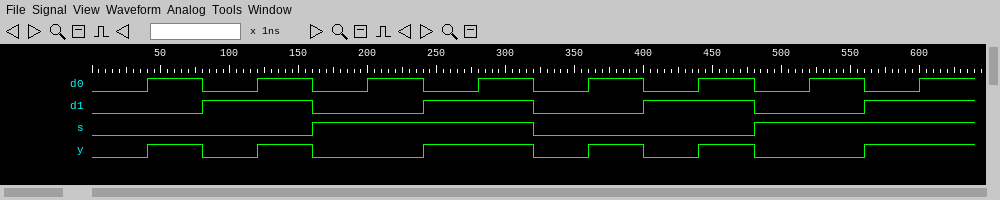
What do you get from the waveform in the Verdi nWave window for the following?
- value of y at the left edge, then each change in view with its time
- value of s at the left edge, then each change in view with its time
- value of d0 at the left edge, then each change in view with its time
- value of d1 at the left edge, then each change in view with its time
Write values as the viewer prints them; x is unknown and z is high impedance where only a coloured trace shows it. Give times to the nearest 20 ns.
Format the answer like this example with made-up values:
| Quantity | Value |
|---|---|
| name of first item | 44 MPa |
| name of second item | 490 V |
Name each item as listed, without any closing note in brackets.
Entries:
| Quantity | Value |
|---|---|
| value of y at the left edge, then each change in view with its time | 0, 1 at 40 ns, 0 at 80 ns, 1 at 120 ns, 0 at 160 ns, 1 at 240 ns, 0 at 320 ns, 1 at 360 ns, 0 at 400 ns, 1 at 440 ns, 0 at 480 ns, 1 at 560 ns |
| value of s at the left edge, then each change in view with its time | 0, 1 at 160 ns, 0 at 320 ns, 1 at 480 ns |
| value of d0 at the left edge, then each change in view with its time | 0, 1 at 40 ns, 0 at 80 ns, 1 at 120 ns, 0 at 160 ns, 1 at 200 ns, 0 at 240 ns, 1 at 280 ns, 0 at 320 ns, 1 at 360 ns, 0 at 400 ns, 1 at 440 ns, 0 at 480 ns, 1 at 520 ns, 0 at 560 ns, 1 at 600 ns |
| value of d1 at the left edge, then each change in view with its time | 0, 1 at 80 ns, 0 at 160 ns, 1 at 240 ns, 0 at 320 ns, 1 at 400 ns, 0 at 480 ns, 1 at 560 ns |
